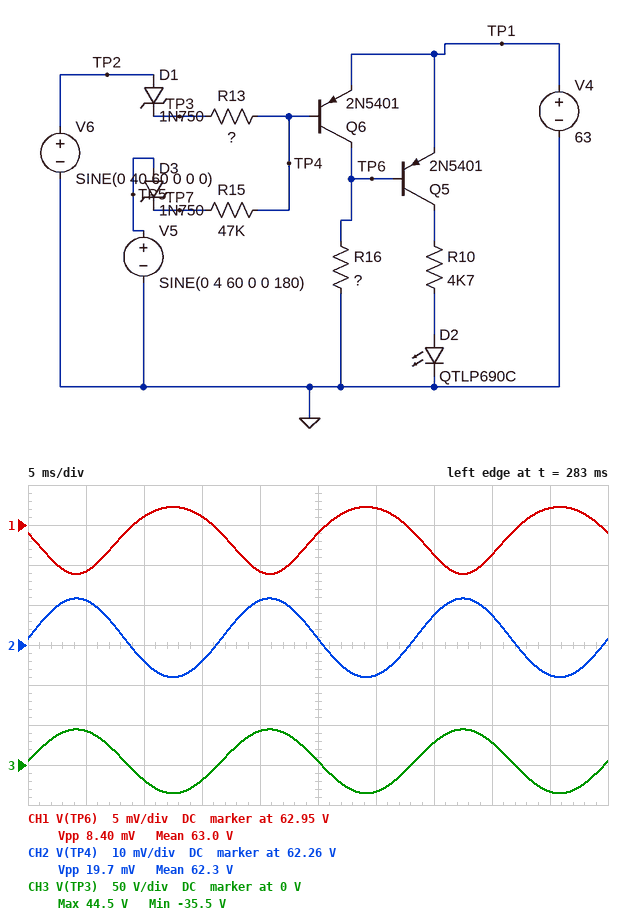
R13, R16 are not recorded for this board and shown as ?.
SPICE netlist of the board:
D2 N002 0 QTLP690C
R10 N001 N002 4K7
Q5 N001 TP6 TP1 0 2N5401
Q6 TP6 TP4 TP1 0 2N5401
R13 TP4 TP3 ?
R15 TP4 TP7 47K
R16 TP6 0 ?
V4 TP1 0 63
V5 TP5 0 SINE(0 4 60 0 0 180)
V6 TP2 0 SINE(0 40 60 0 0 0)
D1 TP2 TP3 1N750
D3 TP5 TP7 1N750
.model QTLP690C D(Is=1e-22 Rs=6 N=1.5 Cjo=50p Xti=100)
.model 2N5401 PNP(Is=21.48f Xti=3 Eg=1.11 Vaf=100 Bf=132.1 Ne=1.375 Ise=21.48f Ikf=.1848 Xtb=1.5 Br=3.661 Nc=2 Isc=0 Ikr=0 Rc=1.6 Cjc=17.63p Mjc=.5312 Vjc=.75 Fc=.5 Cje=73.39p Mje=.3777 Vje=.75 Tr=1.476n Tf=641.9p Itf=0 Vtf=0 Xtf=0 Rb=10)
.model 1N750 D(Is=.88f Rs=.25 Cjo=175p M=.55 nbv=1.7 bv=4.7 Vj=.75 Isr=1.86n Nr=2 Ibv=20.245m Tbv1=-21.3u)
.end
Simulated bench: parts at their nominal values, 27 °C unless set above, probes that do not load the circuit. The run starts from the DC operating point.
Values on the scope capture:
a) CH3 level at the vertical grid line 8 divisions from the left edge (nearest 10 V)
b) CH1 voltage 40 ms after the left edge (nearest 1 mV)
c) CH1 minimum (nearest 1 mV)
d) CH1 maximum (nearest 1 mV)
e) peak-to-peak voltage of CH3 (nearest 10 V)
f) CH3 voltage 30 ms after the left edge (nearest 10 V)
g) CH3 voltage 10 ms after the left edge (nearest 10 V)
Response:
30 V
62.951 V
62.949 V
62.957 V
80 V
-30 V
-20 V
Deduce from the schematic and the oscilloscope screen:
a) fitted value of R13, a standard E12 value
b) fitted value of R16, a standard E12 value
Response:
56 kΩ
5.6 kΩ
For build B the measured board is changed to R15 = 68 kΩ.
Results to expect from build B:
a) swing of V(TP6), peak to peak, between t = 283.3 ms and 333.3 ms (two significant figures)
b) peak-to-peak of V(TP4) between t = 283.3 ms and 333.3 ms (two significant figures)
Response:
12 mV
21 mV
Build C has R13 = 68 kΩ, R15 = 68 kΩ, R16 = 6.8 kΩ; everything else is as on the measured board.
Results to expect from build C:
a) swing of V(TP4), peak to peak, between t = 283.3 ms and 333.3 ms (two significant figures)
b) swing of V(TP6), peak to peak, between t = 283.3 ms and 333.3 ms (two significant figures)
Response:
18 mV
10 mV
